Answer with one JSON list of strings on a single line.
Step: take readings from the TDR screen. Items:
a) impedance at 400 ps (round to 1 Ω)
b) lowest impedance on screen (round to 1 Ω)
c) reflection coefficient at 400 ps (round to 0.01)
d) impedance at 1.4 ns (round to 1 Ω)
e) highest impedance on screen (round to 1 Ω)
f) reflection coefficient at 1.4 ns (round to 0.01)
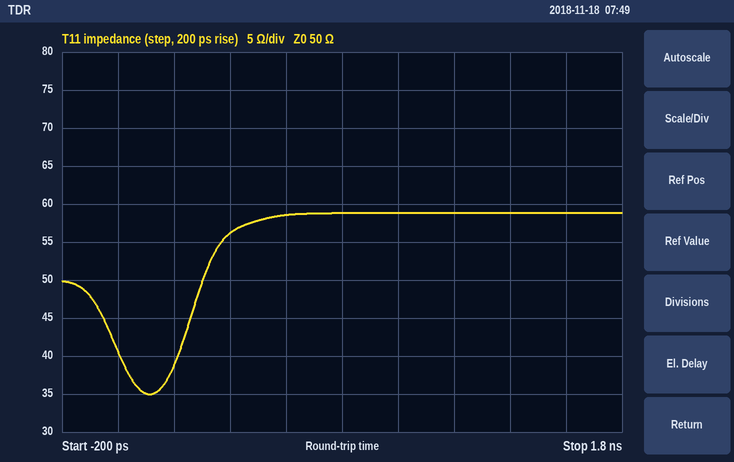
["56 Ω", "35 Ω", "+0.06", "59 Ω", "59 Ω", "+0.08"]
